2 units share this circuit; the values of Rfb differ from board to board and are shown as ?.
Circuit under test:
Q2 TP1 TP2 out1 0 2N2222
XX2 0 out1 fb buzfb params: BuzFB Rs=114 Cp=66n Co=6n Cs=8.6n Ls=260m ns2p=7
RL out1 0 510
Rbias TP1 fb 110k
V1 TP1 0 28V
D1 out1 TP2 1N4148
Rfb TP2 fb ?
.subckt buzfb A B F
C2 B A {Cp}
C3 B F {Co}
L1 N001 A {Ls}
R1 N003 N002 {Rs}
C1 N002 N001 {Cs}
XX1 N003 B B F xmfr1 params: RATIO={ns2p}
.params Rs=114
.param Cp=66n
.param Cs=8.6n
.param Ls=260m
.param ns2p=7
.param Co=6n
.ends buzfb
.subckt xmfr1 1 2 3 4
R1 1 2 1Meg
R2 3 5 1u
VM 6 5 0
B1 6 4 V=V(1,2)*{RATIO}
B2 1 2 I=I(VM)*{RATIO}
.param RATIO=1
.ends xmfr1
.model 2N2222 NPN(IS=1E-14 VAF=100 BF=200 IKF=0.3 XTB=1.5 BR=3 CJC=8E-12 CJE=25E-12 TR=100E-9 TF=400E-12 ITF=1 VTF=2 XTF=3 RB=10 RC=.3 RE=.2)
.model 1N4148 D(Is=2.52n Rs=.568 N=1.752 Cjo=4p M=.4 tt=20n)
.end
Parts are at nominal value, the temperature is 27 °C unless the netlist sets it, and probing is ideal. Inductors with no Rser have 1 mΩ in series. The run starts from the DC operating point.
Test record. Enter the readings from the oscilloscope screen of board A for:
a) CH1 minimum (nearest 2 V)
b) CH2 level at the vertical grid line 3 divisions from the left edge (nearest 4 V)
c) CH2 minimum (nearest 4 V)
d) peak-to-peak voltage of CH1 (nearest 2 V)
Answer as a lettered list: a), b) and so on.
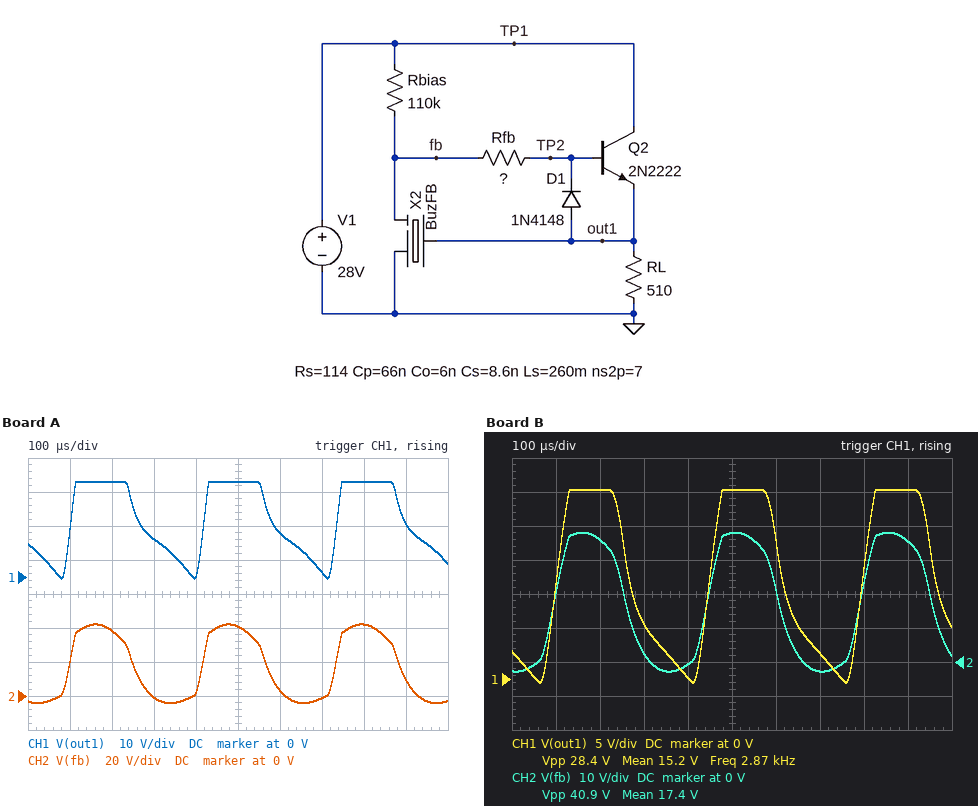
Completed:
a) 0 V
b) 0 V
c) -4 V
d) 28 V
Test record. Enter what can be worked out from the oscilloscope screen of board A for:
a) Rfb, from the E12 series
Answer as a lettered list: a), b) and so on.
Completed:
a) 8.2 kΩ
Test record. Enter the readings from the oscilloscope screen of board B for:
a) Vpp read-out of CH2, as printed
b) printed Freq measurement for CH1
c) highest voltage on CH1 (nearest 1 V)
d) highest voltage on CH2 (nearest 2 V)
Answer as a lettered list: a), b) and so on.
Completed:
a) 40.9 V
b) 2.87 kHz
c) 28 V
d) 38 V
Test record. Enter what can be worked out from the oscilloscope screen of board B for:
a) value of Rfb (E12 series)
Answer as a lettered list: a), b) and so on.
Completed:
a) 15 kΩ
